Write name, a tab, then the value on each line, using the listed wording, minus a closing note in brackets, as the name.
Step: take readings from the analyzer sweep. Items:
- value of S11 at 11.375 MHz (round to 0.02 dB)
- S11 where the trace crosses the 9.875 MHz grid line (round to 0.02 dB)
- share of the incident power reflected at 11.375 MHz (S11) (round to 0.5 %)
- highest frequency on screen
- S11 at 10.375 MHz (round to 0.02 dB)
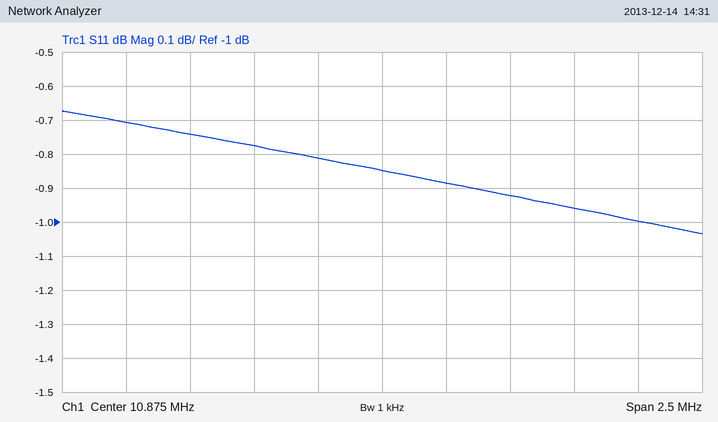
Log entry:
value of S11 at 11.375 MHz	-0.92 dB
S11 where the trace crosses the 9.875 MHz grid line	-0.70 dB
share of the incident power reflected at 11.375 MHz (S11)	81.0 %
highest frequency on screen	12.125 MHz
S11 at 10.375 MHz	-0.78 dB
